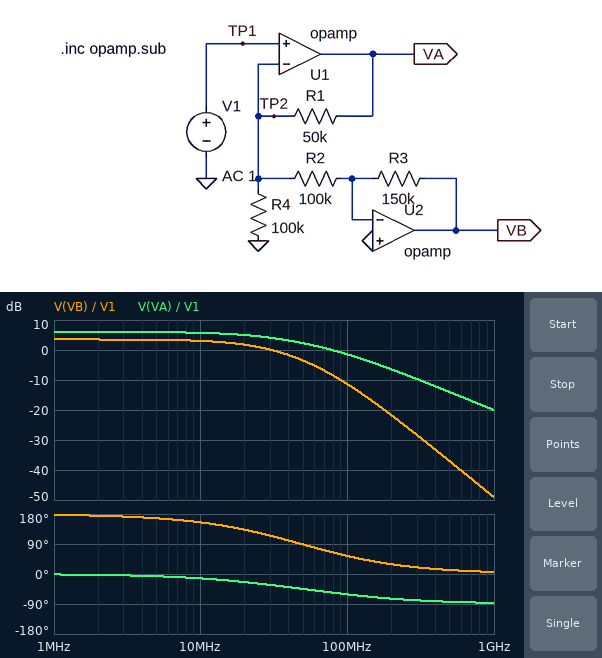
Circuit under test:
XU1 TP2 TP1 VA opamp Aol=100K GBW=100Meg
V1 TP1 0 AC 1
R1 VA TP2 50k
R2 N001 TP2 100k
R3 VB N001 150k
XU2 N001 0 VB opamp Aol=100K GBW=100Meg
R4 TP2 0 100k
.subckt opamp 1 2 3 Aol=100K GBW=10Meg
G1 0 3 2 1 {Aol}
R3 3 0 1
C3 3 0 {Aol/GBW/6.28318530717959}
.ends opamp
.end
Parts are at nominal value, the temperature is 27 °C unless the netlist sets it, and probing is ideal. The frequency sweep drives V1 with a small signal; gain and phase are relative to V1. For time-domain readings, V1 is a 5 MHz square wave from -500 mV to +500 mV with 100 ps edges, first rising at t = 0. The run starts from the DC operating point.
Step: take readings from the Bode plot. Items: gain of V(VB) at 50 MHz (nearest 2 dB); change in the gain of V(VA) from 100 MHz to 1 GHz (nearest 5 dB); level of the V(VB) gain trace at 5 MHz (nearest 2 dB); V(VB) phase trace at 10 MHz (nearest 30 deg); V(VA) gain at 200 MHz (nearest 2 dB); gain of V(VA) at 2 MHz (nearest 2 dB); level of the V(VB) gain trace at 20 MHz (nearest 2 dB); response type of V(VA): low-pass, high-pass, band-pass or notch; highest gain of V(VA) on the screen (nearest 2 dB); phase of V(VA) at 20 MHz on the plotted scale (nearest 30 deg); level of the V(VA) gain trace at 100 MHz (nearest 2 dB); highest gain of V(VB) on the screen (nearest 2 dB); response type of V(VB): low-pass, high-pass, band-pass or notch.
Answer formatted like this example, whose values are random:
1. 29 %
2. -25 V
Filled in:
1. -4 dB
2. -20 dB
3. 4 dB
4. 150 deg
5. -6 dB
6. 6 dB
7. 2 dB
8. low-pass
9. 6 dB
10. -30 deg
11. -2 dB
12. 4 dB
13. low-pass
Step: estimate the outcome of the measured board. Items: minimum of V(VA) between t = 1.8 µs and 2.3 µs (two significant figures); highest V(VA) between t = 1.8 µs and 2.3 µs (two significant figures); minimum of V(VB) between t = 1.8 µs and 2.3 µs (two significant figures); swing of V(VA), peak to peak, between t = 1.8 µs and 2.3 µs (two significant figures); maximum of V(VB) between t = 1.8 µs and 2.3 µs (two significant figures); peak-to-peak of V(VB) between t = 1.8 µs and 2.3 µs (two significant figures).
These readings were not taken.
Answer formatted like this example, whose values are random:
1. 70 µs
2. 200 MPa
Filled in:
1. -1.0 V
2. 1.0 V
3. -750 mV
4. 2.0 V
5. 750 mV
6. 1.5 V
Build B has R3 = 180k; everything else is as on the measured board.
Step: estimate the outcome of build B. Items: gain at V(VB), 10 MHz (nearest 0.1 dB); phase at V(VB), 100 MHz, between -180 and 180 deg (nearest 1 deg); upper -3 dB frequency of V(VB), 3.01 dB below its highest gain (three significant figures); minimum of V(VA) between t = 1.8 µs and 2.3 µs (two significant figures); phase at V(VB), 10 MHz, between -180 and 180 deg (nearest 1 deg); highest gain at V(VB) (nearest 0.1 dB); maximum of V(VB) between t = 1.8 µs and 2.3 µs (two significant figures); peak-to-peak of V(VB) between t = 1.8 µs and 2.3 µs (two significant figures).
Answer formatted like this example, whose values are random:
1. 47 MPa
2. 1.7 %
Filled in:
1. 4.5 dB
2. 52 deg
3. 25.7 MHz
4. -1.0 V
5. 153 deg
6. 5.1 dB
7. 900 mV
8. 1.8 V
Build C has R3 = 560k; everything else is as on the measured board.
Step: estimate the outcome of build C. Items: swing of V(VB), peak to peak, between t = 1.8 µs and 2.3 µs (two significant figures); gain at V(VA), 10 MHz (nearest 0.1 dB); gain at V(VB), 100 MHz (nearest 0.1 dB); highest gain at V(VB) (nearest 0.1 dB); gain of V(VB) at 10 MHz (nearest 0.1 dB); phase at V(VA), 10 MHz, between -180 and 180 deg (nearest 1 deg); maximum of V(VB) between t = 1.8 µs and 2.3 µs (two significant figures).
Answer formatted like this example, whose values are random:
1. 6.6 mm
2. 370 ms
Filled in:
1. 5.6 V
2. 5.2 dB
3. -7.1 dB
4. 15.0 dB
5. 13.1 dB
6. -16 deg
7. 2.8 V
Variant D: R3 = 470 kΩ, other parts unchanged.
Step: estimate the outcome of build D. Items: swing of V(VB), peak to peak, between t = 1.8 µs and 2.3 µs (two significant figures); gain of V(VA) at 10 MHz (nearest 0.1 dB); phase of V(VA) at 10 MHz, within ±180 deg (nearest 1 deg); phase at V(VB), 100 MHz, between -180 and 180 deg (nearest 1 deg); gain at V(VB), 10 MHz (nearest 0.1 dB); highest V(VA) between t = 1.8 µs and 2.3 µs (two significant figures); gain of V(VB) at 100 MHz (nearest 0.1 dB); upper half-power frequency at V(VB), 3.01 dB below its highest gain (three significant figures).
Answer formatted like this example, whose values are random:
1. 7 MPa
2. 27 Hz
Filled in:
1. 4.7 V
2. 5.3 dB
3. -16 deg
4. 44 deg
5. 11.9 dB
6. 1.0 V
7. -7.5 dB
8. 15.2 MHz
